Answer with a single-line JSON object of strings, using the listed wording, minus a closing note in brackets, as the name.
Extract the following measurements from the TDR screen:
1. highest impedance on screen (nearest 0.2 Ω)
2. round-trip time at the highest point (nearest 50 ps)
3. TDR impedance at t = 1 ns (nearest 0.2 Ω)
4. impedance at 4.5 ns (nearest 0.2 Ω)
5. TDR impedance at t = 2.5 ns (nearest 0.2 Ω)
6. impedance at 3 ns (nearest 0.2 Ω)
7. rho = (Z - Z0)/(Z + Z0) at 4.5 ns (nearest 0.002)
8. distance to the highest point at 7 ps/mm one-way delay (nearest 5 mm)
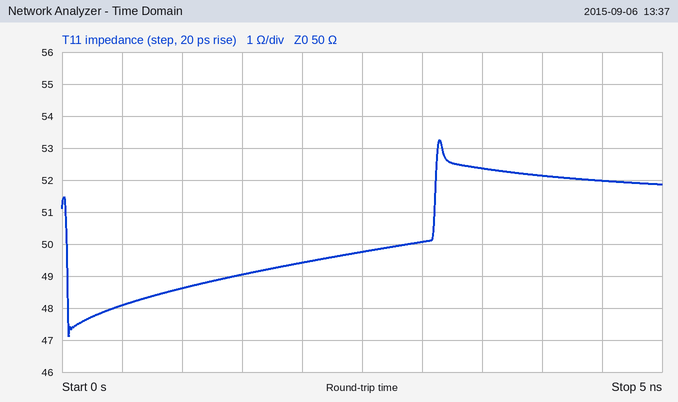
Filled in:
{"highest impedance on screen": "53.2 Ω", "round-trip time at the highest point": "3.15 ns", "TDR impedance at t = 1 ns": "48.6 Ω", "impedance at 4.5 ns": "52.0 Ω", "TDR impedance at t = 2.5 ns": "49.8 Ω", "impedance at 3 ns": "50.0 Ω", "rho = (Z - Z0)/(Z + Z0) at 4.5 ns": "+0.020", "distance to the highest point at 7 ps/mm one-way delay": "225 mm"}
